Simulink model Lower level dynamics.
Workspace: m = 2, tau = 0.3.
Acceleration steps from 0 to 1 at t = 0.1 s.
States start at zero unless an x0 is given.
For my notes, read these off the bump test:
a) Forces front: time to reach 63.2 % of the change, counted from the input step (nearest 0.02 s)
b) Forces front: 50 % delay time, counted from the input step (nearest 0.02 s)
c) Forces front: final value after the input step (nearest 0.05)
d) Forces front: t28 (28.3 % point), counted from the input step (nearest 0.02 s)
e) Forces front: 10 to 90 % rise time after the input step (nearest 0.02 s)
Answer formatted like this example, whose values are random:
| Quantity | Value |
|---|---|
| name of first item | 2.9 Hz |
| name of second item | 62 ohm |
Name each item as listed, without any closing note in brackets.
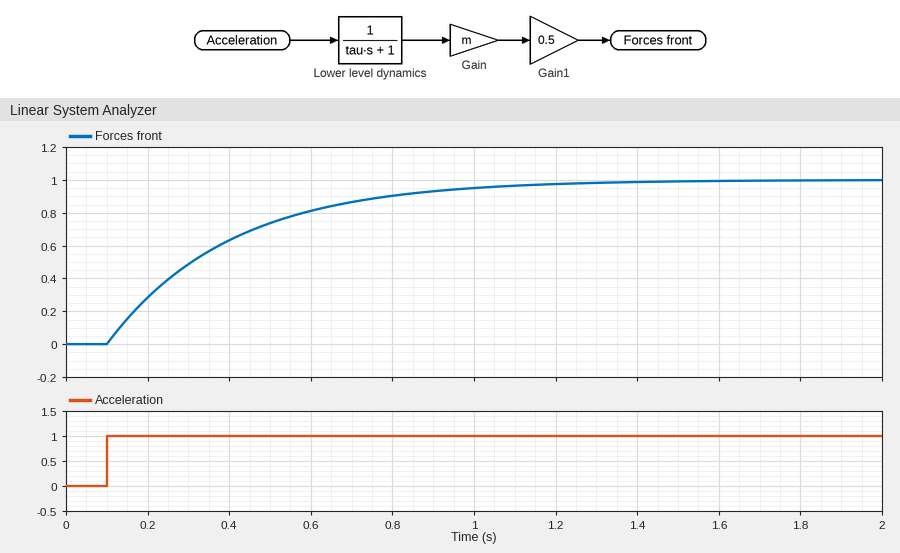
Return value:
| Quantity | Value |
|---|---|
| Forces front: time to reach 63.2 % of the change, counted from the input step | 0.30 s |
| Forces front: 50 % delay time, counted from the input step | 0.20 s |
| Forces front: final value after the input step | 1.00 |
| Forces front: t28 (28.3 % point), counted from the input step | 0.10 s |
| Forces front: 10 to 90 % rise time after the input step | 0.66 s |
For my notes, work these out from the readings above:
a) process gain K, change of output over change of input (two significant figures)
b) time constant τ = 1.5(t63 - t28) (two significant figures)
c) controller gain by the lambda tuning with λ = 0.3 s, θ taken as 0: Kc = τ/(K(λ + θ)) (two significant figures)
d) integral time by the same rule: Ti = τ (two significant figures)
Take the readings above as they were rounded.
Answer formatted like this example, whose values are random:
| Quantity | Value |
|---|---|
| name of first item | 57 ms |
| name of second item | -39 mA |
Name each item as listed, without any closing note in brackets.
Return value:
| Quantity | Value |
|---|---|
| process gain K, change of output over change of input | 1.0 |
| time constant τ = 1.5(t63 - t28) | 0.30 s |
| controller gain by the lambda tuning with λ = 0.3 s, θ taken as 0: Kc = τ/(K(λ + θ)) | 1.0 |
| integral time by the same rule: Ti = τ | 0.30 s |
